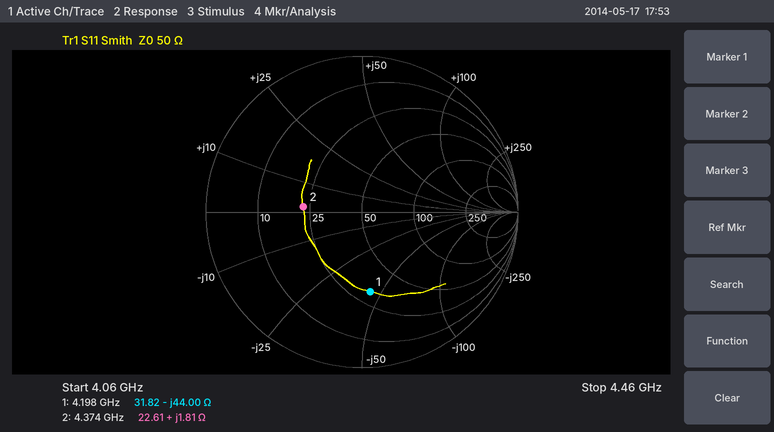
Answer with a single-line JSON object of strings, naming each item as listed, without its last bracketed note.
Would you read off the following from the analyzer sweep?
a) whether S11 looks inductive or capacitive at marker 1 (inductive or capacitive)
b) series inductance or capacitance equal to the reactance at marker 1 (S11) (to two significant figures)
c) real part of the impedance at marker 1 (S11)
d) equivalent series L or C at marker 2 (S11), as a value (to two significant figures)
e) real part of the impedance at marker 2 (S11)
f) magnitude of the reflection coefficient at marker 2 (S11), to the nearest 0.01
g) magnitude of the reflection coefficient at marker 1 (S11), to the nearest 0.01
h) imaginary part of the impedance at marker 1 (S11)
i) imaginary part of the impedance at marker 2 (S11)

{"whether S11 looks inductive or capacitive at marker 1": "capacitive", "series inductance or capacitance equal to the reactance at marker 1 (S11)": "860 fF", "real part of the impedance at marker 1": "31.82 Ω", "equivalent series L or C at marker 2 (S11), as a value": "66 pH", "real part of the impedance at marker 2": "22.61 Ω", "magnitude of the reflection coefficient at marker 2 (S11), to the nearest 0.01": "0.38", "magnitude of the reflection coefficient at marker 1 (S11), to the nearest 0.01": "0.51", "imaginary part of the impedance at marker 1": "-44.00 Ω", "imaginary part of the impedance at marker 2": "+1.81 Ω"}
